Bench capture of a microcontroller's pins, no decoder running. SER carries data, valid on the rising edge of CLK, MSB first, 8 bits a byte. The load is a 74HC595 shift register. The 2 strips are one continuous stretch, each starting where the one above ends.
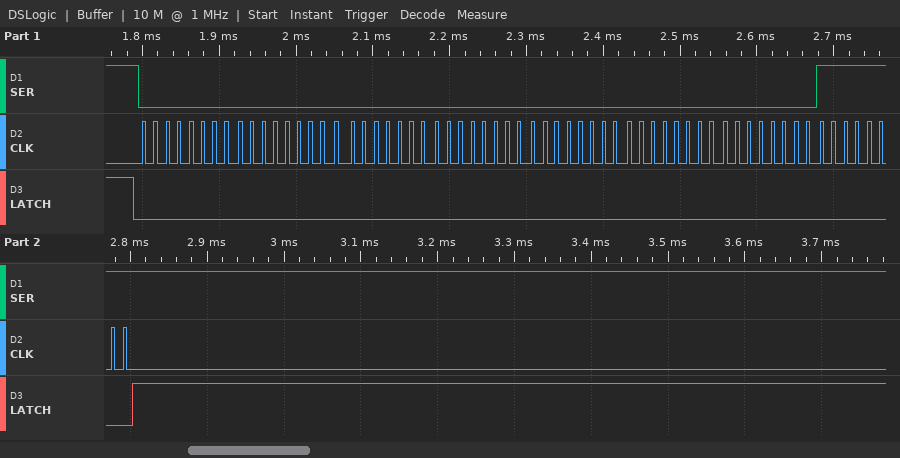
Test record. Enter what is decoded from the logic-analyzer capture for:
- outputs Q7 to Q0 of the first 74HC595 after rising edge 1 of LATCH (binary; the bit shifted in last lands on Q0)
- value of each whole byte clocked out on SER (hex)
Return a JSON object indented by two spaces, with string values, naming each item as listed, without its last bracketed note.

{
  "outputs Q7 to Q0 of the first 74HC595 after rising edge 1 of LATCH": "11111111",
  "value of each whole byte clocked out on SER": "00 00 00 00 00 00 00 FF"
}
